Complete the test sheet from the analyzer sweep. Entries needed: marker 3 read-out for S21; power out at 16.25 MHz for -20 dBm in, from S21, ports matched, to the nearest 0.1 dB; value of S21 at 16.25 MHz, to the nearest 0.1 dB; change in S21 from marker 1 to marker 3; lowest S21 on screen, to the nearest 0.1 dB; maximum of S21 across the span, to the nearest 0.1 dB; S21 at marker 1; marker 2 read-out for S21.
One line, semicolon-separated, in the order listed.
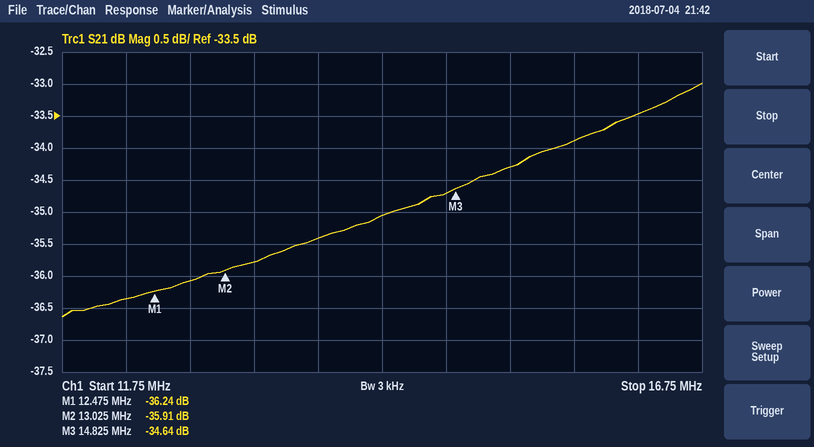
-34.64 dB; -53.5 dBm; -33.5 dB; 1.60 dB; -36.6 dB; -33.0 dB; -36.24 dB; -35.91 dB
